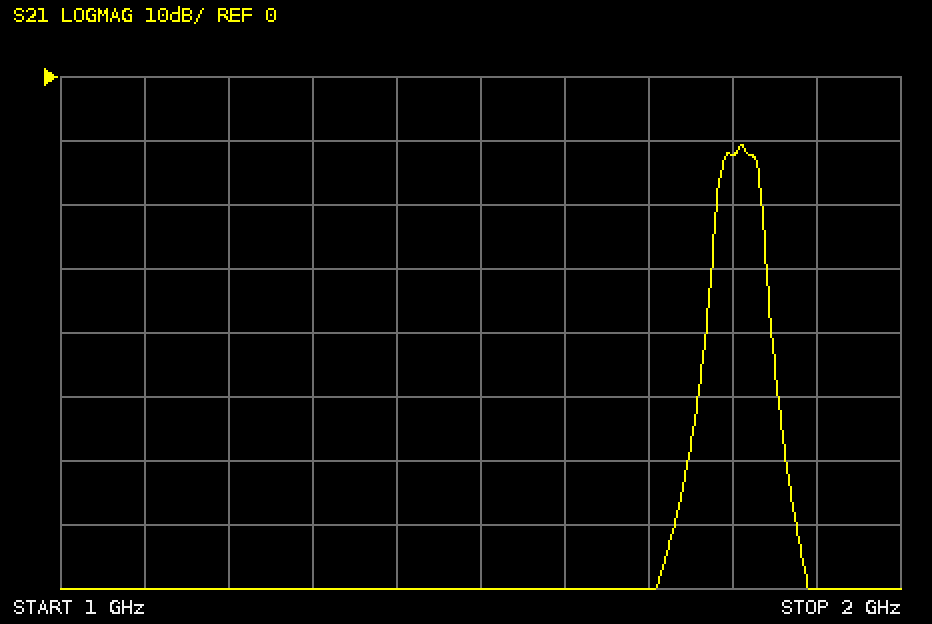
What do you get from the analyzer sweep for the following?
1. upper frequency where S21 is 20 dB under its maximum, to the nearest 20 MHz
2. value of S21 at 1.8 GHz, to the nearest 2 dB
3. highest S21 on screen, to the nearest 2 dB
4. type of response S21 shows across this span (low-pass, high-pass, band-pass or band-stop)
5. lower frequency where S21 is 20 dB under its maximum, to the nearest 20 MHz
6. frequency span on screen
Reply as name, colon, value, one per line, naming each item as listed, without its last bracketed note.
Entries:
upper frequency where S21 is 20 dB under its maximum, to the nearest 20 MHz: 1.84 GHz
value of S21 at 1.8 GHz, to the nearest 2 dB: -12 dB
highest S21 on screen, to the nearest 2 dB: -10 dB
type of response S21 shows across this span: band-pass
lower frequency where S21 is 20 dB under its maximum, to the nearest 20 MHz: 1.78 GHz
frequency span on screen: 1 GHz
